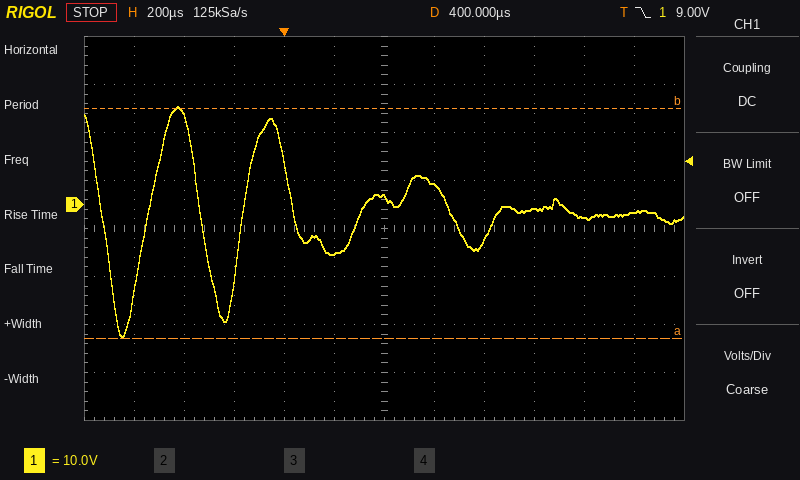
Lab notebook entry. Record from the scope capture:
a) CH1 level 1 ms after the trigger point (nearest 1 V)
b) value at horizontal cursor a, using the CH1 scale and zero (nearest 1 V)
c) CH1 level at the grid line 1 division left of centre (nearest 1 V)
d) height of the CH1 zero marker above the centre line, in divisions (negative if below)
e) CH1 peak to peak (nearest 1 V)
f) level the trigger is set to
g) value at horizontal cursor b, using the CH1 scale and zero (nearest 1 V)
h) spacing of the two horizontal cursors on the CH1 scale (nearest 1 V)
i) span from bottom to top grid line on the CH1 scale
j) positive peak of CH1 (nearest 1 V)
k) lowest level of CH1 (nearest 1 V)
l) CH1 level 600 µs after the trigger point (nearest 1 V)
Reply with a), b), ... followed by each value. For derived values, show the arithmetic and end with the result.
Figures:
a) -1 V
b) -28 V
c) -10 V
d) +0.5 div
e) 20 V − (-28 V) = 48 V
f) 9.00 V
g) 20 V
h) 48 V
i) 80 V
j) 20 V
k) -28 V
l) 4 V
